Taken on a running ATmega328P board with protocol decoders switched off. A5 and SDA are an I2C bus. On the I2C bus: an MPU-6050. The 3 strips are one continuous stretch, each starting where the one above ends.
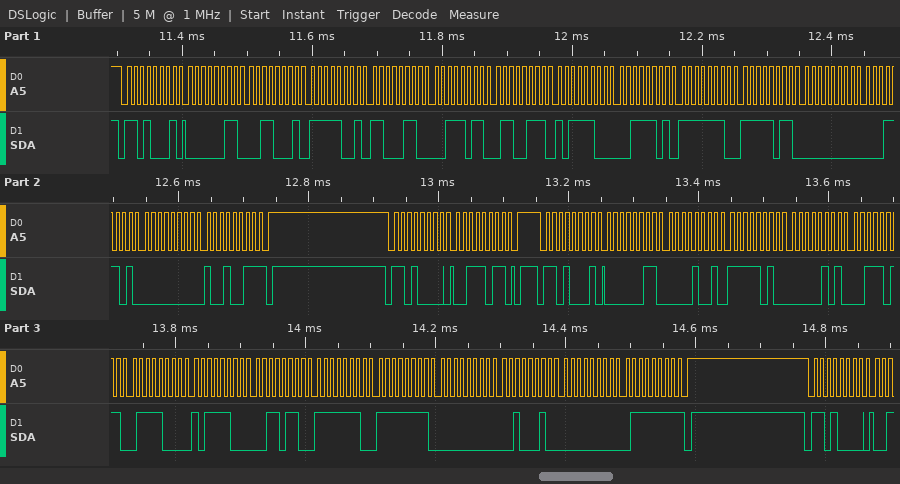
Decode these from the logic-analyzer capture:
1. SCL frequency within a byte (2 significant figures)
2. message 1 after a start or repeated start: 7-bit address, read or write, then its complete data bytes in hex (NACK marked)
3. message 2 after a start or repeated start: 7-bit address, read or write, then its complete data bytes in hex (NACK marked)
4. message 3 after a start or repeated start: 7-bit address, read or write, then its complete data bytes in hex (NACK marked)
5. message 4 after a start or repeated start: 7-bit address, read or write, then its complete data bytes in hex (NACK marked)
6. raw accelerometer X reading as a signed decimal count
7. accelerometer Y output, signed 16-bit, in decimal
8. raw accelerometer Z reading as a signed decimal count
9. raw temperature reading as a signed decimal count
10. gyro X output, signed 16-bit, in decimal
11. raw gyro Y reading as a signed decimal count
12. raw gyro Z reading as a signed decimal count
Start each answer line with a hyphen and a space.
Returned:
- 100 kHz
- 0x68 read: 03 31 F9 C6 3B 67 BC 3D FE FB 00 1D 00 93 NACK
- 0x68 write: 3B
- 0x68 read: 03 09 FA 05 3B 78 BC 36 FE FF 00 22 00 7F NACK
- 0x68 write
- 777
- -1531
- 15224
- -17354
- -257
- 34
- 127
